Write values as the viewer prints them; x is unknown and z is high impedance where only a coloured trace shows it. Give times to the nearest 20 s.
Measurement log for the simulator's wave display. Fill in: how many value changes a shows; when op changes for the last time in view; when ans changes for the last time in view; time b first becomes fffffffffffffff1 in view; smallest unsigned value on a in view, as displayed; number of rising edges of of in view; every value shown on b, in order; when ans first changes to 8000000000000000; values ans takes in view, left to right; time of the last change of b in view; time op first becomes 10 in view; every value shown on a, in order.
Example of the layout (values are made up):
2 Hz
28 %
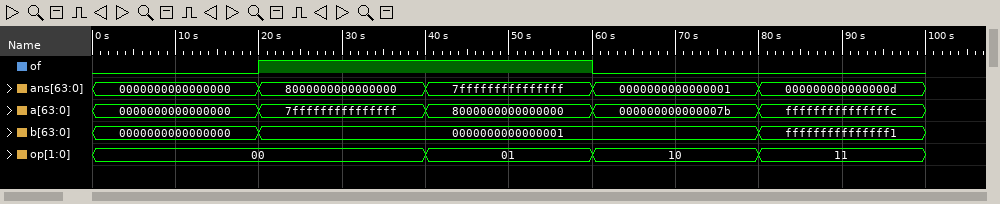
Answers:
4
80 s
80 s
80 s
0000000000000000
1
0000000000000000, 0000000000000001, fffffffffffffff1
20 s
0000000000000000, 8000000000000000, 7fffffffffffffff, 0000000000000001, 000000000000000d
80 s
60 s
0000000000000000, 7fffffffffffffff, 8000000000000000, 000000000000007b, fffffffffffffffc
